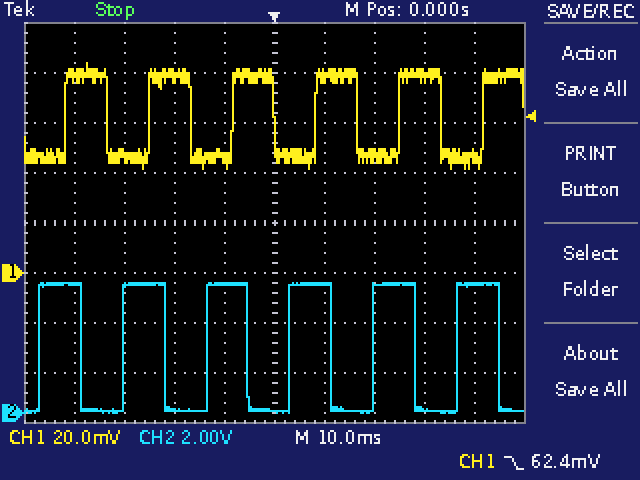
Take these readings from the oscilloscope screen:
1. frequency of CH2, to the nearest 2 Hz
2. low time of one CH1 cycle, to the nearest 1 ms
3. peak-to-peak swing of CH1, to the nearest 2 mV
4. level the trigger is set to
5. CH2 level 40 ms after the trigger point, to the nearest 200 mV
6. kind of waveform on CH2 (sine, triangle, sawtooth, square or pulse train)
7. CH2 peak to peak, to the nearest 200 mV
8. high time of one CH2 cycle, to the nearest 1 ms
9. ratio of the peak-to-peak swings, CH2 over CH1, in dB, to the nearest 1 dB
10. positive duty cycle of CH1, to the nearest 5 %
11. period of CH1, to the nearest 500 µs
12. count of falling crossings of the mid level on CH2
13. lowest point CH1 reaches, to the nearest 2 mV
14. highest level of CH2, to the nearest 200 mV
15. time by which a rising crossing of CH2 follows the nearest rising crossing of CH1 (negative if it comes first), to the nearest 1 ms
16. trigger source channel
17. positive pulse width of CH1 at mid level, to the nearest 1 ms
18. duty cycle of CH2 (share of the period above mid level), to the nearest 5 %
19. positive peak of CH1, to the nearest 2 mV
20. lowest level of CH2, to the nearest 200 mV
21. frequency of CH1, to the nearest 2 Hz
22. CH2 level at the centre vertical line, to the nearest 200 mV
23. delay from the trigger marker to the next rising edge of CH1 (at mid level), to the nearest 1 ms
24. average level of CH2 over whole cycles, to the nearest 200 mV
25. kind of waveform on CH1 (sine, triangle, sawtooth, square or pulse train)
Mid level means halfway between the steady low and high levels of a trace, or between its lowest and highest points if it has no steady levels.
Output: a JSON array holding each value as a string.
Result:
["60 Hz", "8 ms", "42 mV", "62.4 mV", "5.2 V", "square", "5.2 V", "8 ms", "42 dB", "50 %", "16.5 ms", "6", "42 mV", "5.2 V", "-5 ms", "CH1", "8 ms", "50 %", "84 mV", "0.0 V", "60 Hz", "0.0 V", "8 ms", "2.6 V", "square"]
